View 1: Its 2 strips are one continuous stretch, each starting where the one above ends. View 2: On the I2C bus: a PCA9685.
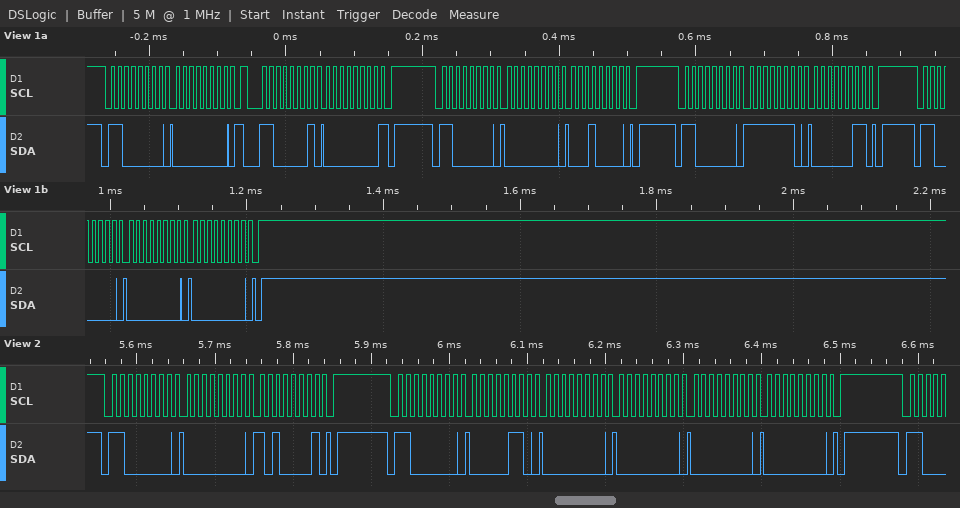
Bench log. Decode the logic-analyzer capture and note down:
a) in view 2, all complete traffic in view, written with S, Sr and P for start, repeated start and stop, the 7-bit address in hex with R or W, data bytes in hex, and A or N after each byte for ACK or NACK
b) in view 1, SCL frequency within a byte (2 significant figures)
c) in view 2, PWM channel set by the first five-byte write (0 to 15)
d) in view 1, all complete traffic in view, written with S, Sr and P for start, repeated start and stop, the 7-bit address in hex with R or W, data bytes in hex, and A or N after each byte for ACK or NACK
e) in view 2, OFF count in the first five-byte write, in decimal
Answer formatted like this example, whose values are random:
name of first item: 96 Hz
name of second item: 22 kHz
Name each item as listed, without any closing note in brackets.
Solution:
in view 2, all complete traffic in view, written with S, Sr and P for start, repeated start and stop, the 7-bit address in hex with R or W, data bytes in hex, and A or N after each byte for ACK or NACK: S 60W A 00 A A1 A P S 60W A 06 A 00 A 00 A 00 A 00 A P
in view 1, SCL frequency within a byte: 100 kHz
in view 2, PWM channel set by the first five-byte write: 0
in view 1, all complete traffic in view, written with S, Sr and P for start, repeated start and stop, the 7-bit address in hex with R or W, data bytes in hex, and A or N after each byte for ACK or NACK: S 60W A 00 A Sr 60R A 00 N P S 60W A 00 A 10 A P S 60W A FE A 03 A P S 60W A 00 A 00 A P
in view 2, OFF count in the first five-byte write, in decimal: 0
